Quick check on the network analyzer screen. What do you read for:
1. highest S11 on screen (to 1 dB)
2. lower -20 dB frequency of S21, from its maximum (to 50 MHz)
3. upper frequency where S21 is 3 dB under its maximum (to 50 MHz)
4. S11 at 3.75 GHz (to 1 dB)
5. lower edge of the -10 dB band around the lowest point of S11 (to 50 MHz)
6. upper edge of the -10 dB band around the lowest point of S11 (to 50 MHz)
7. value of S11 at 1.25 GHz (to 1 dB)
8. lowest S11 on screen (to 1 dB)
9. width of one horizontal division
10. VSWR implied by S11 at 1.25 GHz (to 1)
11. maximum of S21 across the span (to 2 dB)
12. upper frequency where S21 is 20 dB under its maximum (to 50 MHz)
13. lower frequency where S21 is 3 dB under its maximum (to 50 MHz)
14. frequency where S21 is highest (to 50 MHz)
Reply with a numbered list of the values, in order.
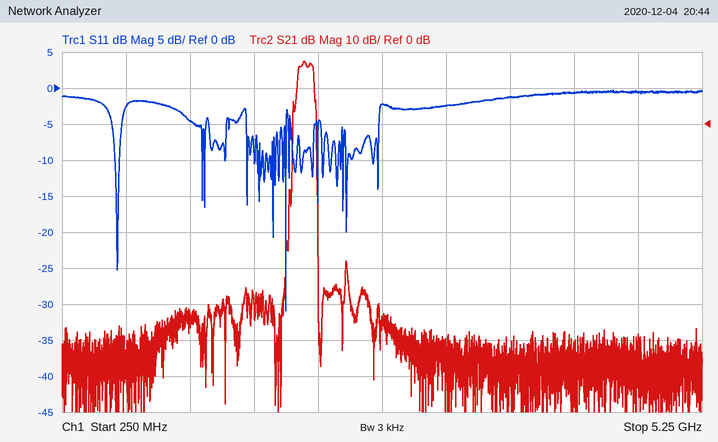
1. 0 dB
2. 2.05 GHz
3. 2.20 GHz
4. -1 dB
5. 2.00 GHz
6. 2.00 GHz
7. -5 dB
8. -31 dB
9. 500 MHz
10. 4
11. 18 dB
12. 2.25 GHz
13. 2.10 GHz
14. 2.15 GHz
